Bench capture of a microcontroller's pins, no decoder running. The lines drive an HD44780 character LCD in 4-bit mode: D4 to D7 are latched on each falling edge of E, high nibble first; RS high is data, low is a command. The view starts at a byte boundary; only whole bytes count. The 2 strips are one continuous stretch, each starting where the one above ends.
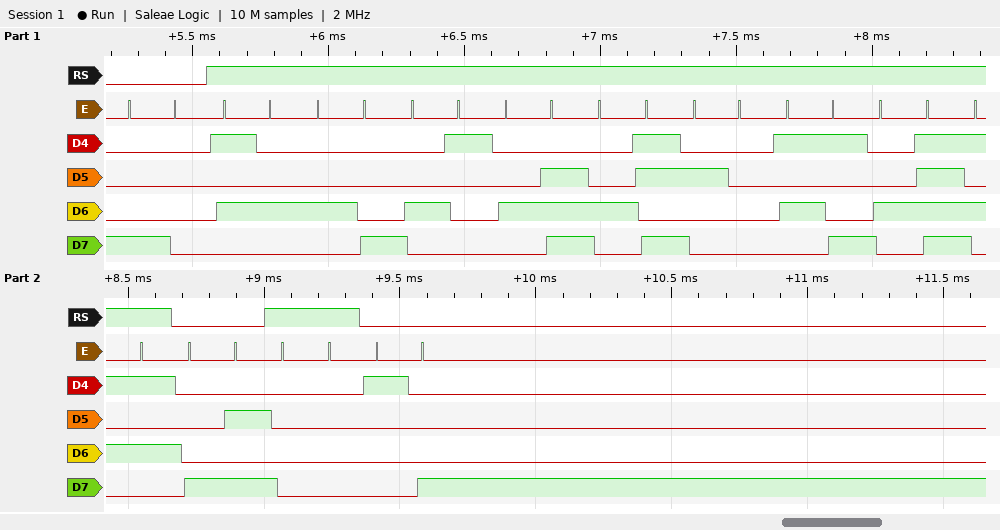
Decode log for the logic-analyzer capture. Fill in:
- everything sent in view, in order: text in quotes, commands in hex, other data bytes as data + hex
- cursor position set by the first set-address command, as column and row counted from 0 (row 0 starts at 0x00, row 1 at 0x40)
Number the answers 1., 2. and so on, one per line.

1. 0x80 "THANK YOU" 0x8A data 00 0x18
2. column 0, row 0
